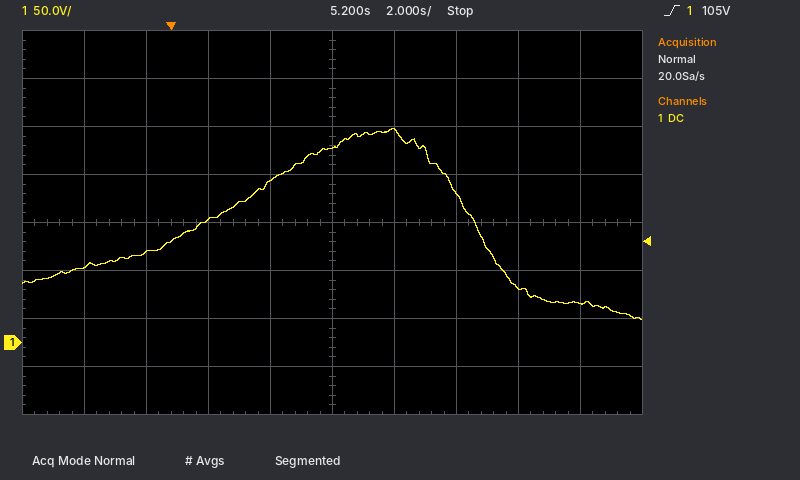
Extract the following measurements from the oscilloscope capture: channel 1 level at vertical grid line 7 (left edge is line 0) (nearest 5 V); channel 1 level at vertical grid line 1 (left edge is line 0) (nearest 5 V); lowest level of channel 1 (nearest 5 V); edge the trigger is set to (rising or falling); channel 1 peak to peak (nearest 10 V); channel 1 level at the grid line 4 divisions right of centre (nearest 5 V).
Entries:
155 V
80 V
25 V
rising
200 V
40 V
